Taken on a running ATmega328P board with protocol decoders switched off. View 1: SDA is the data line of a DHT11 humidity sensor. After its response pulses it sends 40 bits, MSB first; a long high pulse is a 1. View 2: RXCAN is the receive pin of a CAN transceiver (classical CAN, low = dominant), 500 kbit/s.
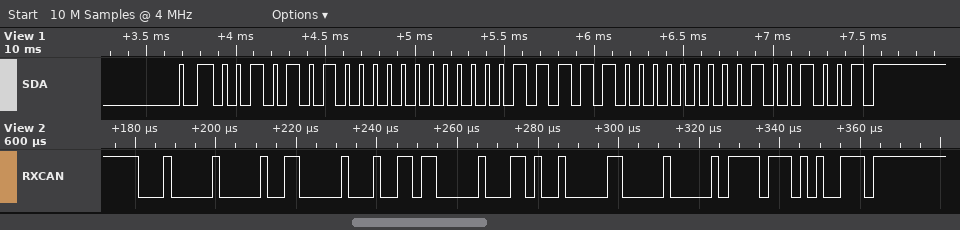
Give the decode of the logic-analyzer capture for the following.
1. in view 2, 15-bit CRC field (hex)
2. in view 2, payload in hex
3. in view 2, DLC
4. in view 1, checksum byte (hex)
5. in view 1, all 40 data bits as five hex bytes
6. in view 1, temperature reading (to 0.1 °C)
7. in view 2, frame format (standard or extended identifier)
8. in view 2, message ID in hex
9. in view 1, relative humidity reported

0x7753
01 36 01 A4 10 01
6
0x49
2A 00 1F 00 49
31.0 °C
standard
0x100
42 %
